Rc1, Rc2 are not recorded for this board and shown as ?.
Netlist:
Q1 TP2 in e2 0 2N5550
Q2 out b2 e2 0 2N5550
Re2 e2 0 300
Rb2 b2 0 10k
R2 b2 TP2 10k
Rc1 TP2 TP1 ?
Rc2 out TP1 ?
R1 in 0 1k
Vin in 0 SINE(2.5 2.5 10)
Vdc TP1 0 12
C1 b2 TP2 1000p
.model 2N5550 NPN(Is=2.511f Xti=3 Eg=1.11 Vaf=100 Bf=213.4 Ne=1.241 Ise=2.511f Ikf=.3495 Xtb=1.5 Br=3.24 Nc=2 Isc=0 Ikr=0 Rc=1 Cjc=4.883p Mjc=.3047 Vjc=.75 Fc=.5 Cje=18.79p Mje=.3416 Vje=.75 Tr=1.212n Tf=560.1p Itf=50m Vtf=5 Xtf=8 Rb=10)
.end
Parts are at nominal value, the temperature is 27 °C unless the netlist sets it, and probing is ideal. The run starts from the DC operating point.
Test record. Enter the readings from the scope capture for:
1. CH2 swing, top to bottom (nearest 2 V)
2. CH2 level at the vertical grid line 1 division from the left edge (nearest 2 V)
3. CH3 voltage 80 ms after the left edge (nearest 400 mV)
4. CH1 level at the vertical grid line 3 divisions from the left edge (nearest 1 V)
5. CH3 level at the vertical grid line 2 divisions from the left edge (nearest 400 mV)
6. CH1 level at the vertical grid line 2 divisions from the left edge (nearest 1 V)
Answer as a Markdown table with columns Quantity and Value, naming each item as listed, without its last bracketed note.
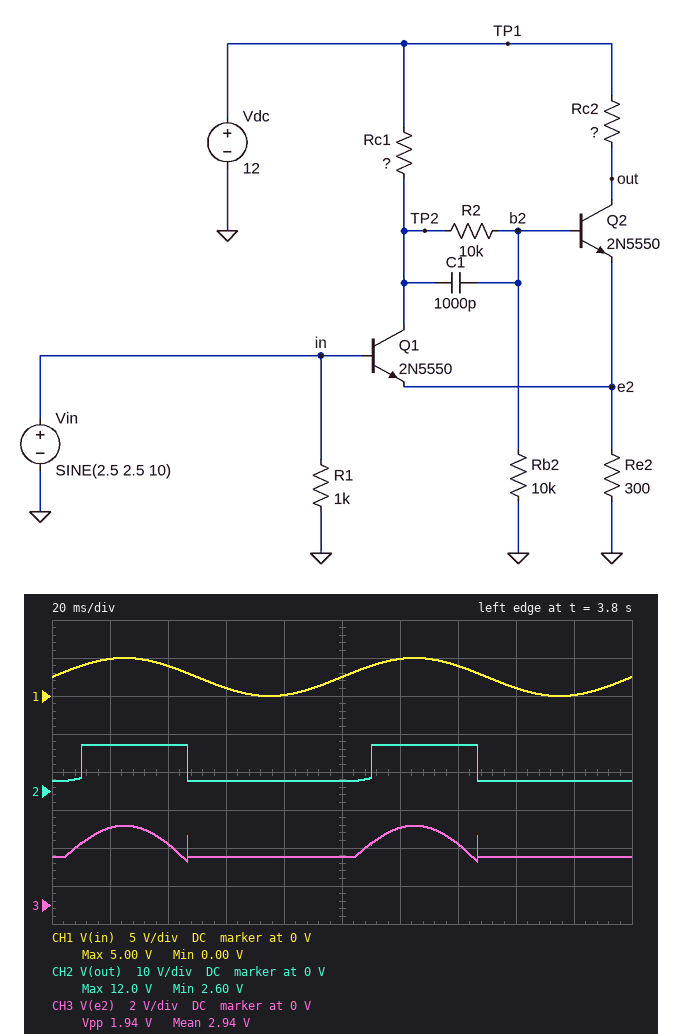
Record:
| Quantity | Value |
|---|---|
| CH2 swing, top to bottom | 10 V |
| CH2 level at the vertical grid line 1 division from the left edge | 12 V |
| CH3 voltage 80 ms after the left edge | 2.4 V |
| CH1 level at the vertical grid line 3 divisions from the left edge | 1 V |
| CH3 level at the vertical grid line 2 divisions from the left edge | 3.2 V |
| CH1 level at the vertical grid line 2 divisions from the left edge | 4 V |
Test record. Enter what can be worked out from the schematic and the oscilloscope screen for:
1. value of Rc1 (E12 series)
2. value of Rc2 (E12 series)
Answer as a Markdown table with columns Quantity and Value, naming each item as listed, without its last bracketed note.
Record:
| Quantity | Value |
|---|---|
| value of Rc1 | 820 Ω |
| value of Rc2 | 1.2 kΩ |
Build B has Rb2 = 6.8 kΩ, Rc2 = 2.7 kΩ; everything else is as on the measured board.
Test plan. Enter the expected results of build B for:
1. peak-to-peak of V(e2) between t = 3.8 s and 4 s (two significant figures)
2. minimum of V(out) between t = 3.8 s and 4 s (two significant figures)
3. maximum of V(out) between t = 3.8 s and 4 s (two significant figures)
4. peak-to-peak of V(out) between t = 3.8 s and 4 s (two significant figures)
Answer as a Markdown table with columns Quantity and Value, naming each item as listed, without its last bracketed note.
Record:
| Quantity | Value |
|---|---|
| peak-to-peak of V(e2) between t = 3.8 s and 4 s | 2.8 V |
| minimum of V(out) between t = 3.8 s and 4 s | 1.4 V |
| maximum of V(out) between t = 3.8 s and 4 s | 12 V |
| peak-to-peak of V(out) between t = 3.8 s and 4 s | 11 V |
